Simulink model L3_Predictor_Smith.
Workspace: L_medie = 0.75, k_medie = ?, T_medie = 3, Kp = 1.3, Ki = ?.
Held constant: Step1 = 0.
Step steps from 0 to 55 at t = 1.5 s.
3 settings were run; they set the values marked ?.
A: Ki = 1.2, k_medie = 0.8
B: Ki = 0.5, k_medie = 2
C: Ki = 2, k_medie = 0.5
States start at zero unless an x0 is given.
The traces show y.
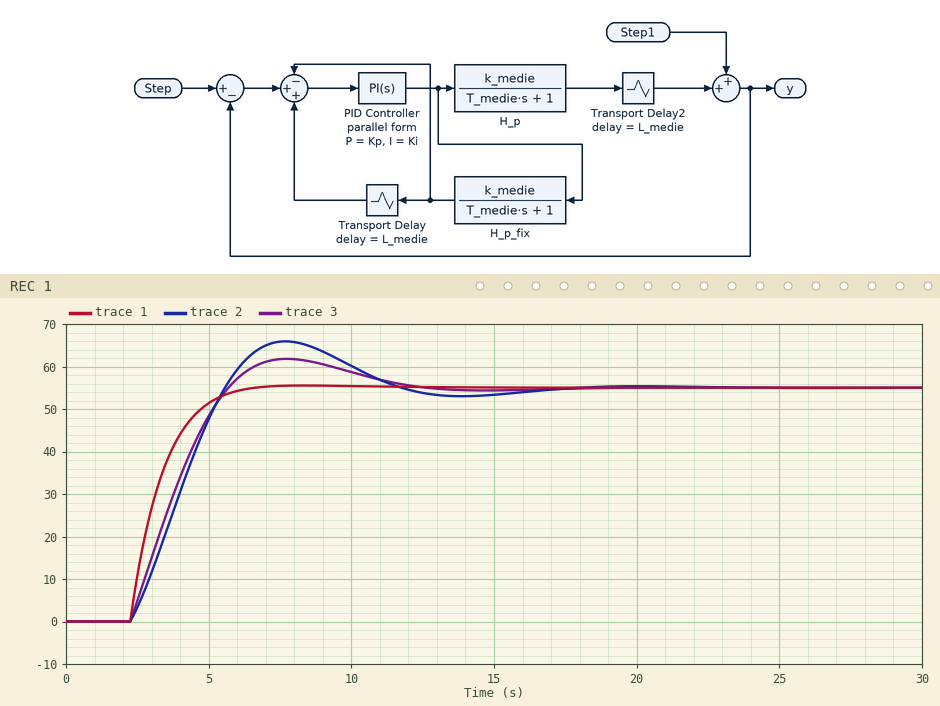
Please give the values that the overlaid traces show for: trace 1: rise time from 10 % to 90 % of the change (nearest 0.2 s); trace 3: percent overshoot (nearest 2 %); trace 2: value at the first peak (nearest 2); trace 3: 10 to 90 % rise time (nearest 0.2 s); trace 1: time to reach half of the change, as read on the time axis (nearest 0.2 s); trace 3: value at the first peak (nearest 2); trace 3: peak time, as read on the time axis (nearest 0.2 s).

2.2 s
12 %
66
2.6 s
3.0 s
62
7.8 s
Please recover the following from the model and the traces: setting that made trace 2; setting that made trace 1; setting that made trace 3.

C
B
A
